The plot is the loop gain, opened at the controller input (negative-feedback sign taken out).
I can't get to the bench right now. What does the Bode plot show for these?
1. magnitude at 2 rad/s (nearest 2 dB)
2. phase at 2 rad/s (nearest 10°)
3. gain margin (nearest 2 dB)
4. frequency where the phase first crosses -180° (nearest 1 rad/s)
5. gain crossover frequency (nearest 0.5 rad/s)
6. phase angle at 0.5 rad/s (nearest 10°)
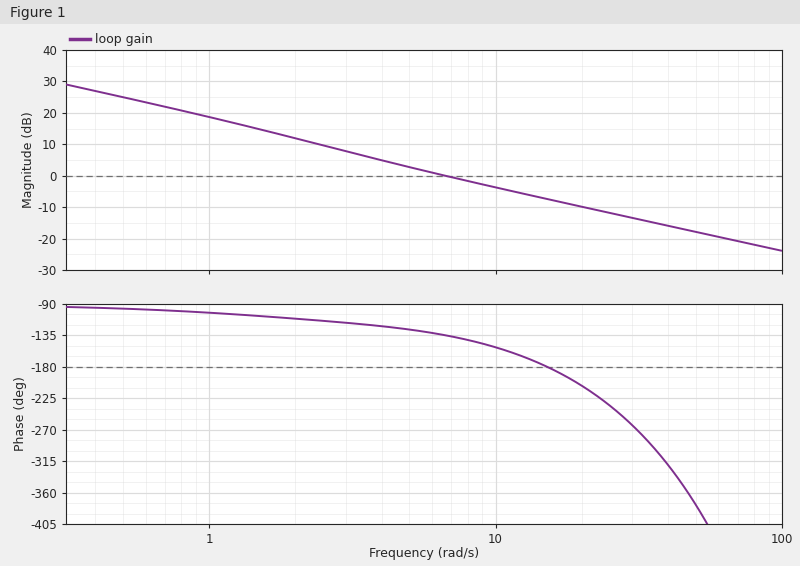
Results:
12 dB
-110°
8 dB
15 rad/s
6.5 rad/s
-100°
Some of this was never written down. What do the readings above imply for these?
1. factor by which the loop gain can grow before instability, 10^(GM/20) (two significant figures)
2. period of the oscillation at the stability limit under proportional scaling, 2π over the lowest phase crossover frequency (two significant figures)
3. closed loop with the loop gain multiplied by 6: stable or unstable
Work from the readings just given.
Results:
2.5
0.42 s
unstable
